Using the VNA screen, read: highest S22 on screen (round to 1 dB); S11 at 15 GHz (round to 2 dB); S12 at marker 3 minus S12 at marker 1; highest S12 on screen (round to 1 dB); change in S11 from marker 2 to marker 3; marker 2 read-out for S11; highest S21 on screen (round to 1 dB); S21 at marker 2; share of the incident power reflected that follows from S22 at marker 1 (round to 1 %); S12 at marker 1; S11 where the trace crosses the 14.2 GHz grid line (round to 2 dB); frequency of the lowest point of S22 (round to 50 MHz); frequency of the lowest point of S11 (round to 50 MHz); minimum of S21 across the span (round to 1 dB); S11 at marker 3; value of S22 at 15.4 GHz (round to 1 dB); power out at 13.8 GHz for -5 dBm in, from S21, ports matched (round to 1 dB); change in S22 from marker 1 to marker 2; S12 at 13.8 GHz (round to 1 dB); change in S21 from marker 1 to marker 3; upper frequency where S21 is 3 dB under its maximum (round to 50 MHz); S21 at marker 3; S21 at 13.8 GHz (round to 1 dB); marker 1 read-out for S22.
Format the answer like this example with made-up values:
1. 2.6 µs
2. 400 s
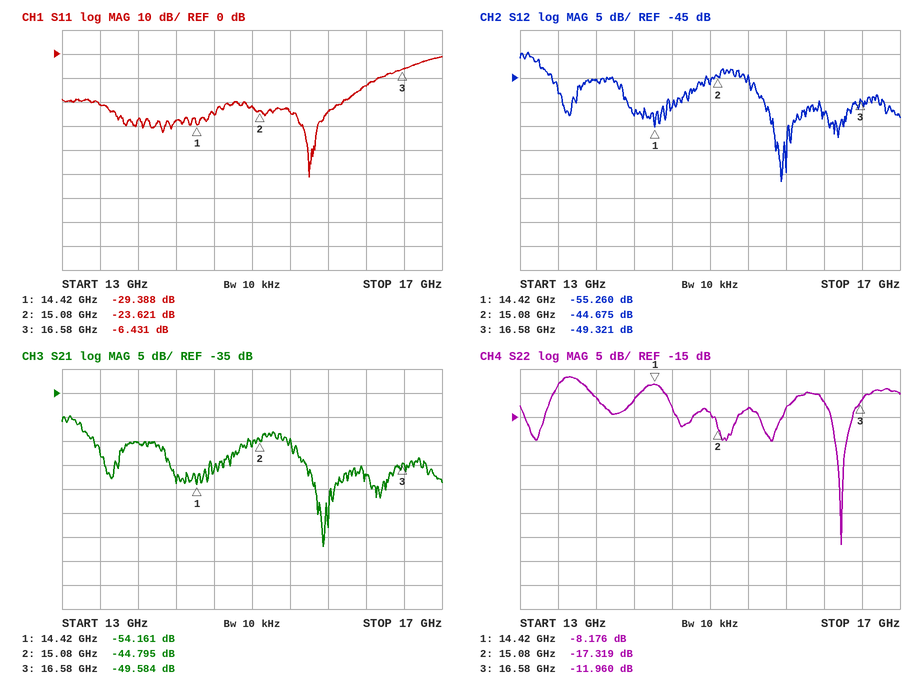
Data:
1. -7 dB
2. -22 dB
3. 5.939 dB
4. -40 dB
5. 17.190 dB
6. -23.621 dB
7. -40 dB
8. -44.795 dB
9. 15 %
10. -55.260 dB
11. -28 dB
12. 16.40 GHz
13. 15.60 GHz
14. -67 dB
15. -6.431 dB
16. -13 dB
17. -50 dBm
18. -9.143 dB
19. -45 dB
20. 4.577 dB
21. 13.20 GHz
22. -49.584 dB
23. -45 dB
24. -8.176 dB
